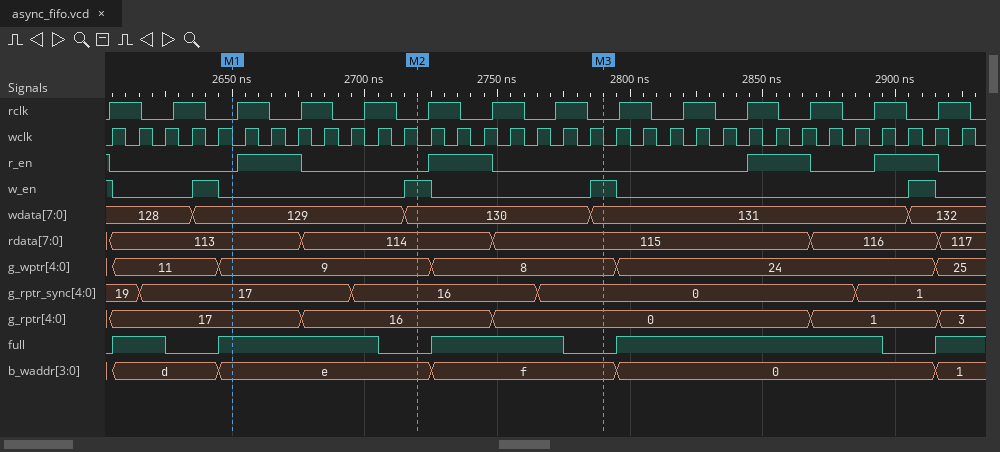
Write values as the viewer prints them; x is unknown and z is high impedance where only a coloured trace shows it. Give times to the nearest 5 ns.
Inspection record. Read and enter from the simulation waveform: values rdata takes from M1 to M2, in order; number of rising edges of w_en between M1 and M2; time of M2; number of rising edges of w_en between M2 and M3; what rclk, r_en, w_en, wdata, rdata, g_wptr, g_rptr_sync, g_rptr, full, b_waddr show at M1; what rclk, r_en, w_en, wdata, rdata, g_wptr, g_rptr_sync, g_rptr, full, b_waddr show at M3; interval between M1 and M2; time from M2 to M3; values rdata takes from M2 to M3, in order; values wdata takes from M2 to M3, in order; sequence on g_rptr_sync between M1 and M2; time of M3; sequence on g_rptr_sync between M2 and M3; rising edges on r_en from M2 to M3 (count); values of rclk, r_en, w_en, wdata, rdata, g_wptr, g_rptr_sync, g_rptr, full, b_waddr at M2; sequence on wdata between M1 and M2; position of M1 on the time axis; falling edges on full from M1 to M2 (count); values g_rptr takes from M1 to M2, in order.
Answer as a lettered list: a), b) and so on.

a) 113, 114
b) 1
c) 2720 ns
d) 1
e) rclk=0, r_en=0, w_en=0, wdata=129, rdata=113, g_wptr=9, g_rptr_sync=17, g_rptr=17, full=1, b_waddr=e
f) rclk=0, r_en=0, w_en=1, wdata=131, rdata=115, g_wptr=8, g_rptr_sync=0, g_rptr=0, full=0, b_waddr=f
g) 70 ns
h) 70 ns
i) 114, 115
j) 130, 131
k) 17, 16
l) 2790 ns
m) 16, 0
n) 1
o) rclk=0, r_en=0, w_en=1, wdata=130, rdata=114, g_wptr=9, g_rptr_sync=16, g_rptr=16, full=0, b_waddr=e
p) 129, 130
q) 2650 ns
r) 1
s) 17, 16
